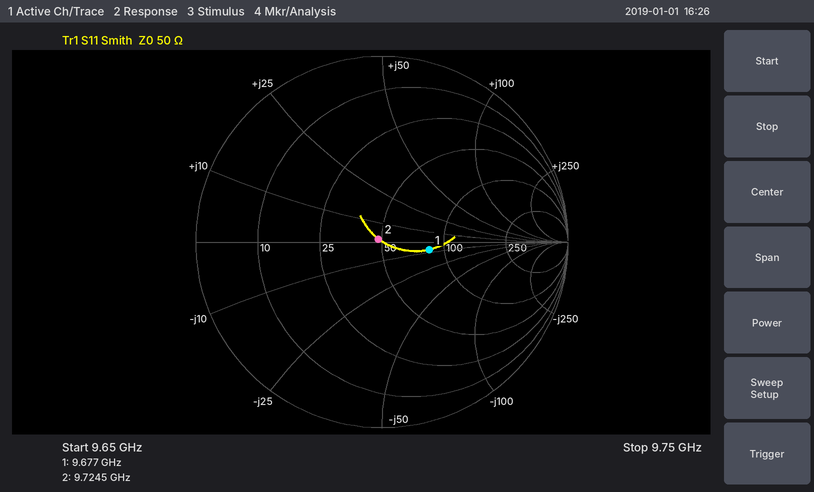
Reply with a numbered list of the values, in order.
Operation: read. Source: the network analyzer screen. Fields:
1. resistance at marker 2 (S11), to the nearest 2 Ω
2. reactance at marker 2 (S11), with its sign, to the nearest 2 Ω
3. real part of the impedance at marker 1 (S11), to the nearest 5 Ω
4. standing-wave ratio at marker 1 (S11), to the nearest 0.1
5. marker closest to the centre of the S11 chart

1. 48 Ω
2. +2 Ω
3. 85 Ω
4. 1.7
5. marker 2
